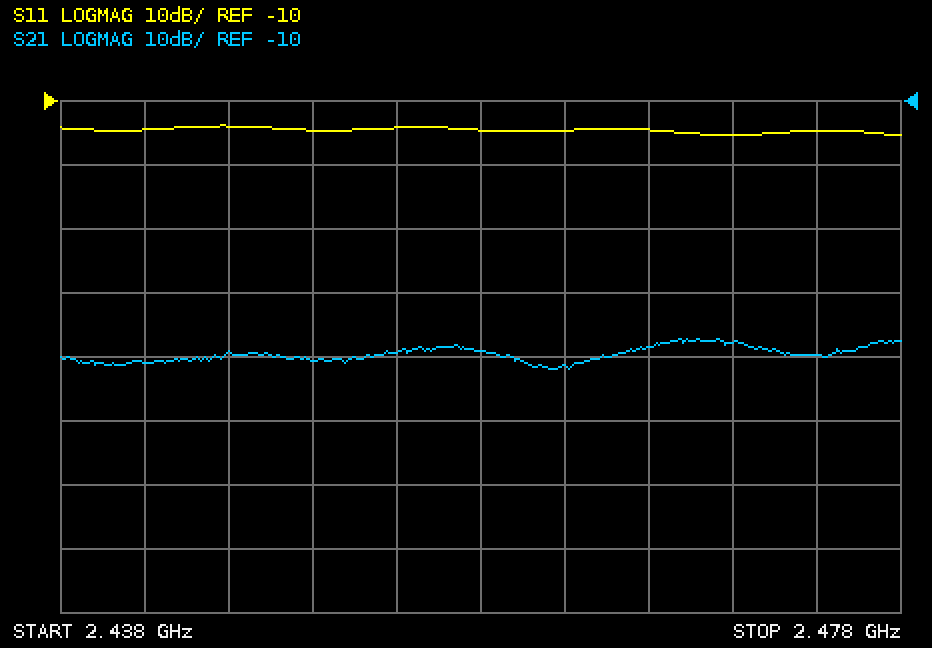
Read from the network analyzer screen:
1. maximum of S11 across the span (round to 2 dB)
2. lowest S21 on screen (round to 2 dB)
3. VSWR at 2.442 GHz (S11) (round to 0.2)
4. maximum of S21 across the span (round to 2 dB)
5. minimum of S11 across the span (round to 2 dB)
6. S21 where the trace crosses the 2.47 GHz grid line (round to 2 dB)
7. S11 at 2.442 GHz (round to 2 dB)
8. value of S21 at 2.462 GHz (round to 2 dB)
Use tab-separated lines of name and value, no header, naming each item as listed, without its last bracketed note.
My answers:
maximum of S11 across the span	-14 dB
lowest S21 on screen	-52 dB
VSWR at 2.442 GHz (S11)	1.4
maximum of S21 across the span	-48 dB
minimum of S11 across the span	-16 dB
S21 where the trace crosses the 2.47 GHz grid line	-48 dB
S11 at 2.442 GHz	-14 dB
value of S21 at 2.462 GHz	-52 dB
